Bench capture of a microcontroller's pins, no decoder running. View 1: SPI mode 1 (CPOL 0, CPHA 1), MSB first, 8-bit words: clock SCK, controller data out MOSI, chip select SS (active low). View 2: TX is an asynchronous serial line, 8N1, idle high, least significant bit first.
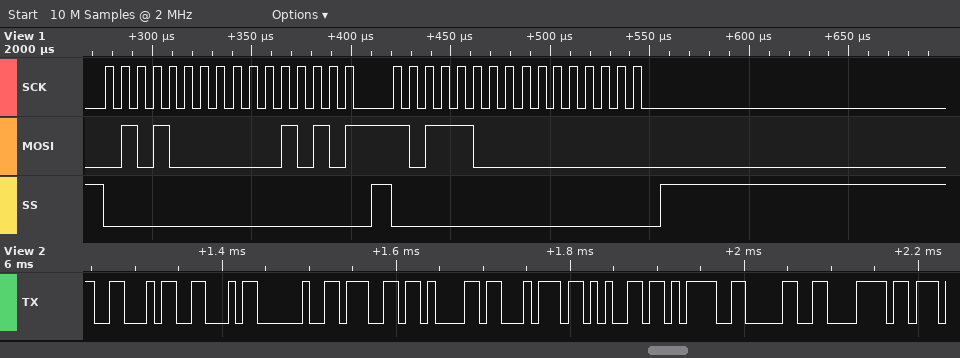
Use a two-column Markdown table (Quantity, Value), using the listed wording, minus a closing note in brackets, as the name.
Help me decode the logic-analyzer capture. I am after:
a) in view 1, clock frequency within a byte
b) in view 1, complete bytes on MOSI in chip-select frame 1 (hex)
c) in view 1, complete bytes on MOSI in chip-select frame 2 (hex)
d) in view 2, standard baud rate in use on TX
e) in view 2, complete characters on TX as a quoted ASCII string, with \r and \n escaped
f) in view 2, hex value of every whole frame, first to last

| Quantity | Value |
|---|---|
| in view 1, clock frequency within a byte | 125 kHz |
| in view 1, complete bytes on MOSI in chip-select frame 1 | 50 15 |
| in view 1, complete bytes on MOSI in chip-select frame 2 | B8 00 |
| in view 2, standard baud rate in use on TX | 115200 baud |
| in view 2, complete characters on TX as a quoted ASCII string, with \r and \n escaped | "FF gate=0x" |
| in view 2, hex value of every whole frame, first to last | 0x46 0x46 0x20 0x67 0x61 0x74 0x65 0x3D 0x30 0x78 |
